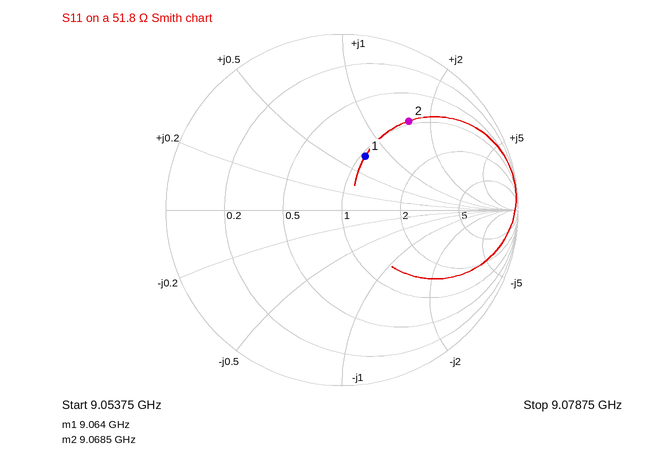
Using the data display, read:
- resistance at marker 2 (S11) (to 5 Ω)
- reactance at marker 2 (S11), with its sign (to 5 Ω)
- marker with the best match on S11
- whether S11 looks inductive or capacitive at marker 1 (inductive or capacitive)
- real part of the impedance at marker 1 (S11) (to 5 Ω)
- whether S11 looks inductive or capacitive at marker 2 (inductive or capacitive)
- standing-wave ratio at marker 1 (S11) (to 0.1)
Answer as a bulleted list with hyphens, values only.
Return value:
- 50 Ω
- +80 Ω
- marker 1
- inductive
- 55 Ω
- inductive
- 2.0
